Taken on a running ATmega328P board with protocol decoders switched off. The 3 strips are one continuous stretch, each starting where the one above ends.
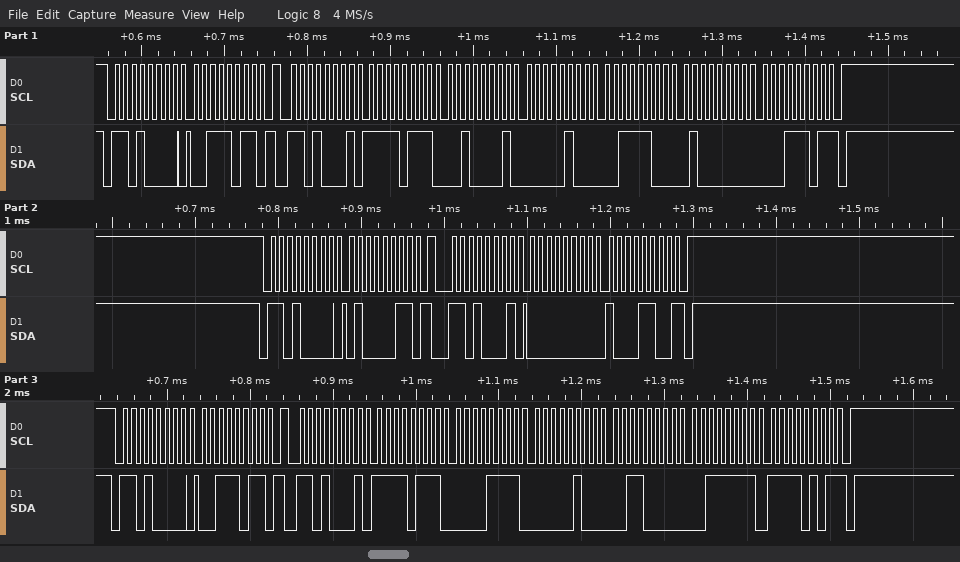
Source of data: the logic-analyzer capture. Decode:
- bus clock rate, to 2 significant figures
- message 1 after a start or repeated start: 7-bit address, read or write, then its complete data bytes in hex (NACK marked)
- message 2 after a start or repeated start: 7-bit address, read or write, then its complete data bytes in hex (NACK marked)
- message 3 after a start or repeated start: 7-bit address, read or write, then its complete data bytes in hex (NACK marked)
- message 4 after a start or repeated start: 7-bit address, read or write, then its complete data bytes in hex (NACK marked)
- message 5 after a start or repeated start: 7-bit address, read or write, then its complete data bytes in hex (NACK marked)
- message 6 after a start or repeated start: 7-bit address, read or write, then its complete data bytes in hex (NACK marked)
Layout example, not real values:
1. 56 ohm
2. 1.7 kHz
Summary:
1. 100 kHz
2. 0x68 write: 3B
3. 0x68 read: F7 21 04 3C 40 1D NACK
4. 0x68 write: 43
5. 0x68 read: 00 8C NACK
6. 0x68 write: 3B
7. 0x68 read: F7 0F 04 30 3F F5 NACK
